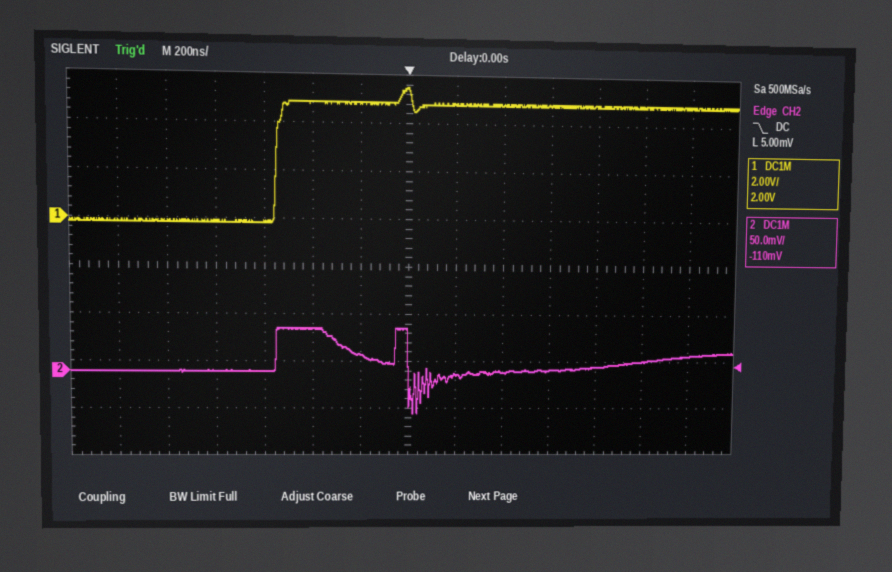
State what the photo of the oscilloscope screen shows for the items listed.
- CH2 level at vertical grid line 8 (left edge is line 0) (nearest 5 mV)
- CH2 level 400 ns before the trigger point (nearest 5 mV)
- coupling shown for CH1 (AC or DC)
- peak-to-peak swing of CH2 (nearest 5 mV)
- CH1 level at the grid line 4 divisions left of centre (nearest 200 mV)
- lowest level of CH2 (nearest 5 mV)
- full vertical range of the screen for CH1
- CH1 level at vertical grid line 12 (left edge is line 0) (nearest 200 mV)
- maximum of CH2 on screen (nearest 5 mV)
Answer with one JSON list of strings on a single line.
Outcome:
["-5 mV", "45 mV", "DC", "90 mV", "-200 mV", "-45 mV", "16 V", "4.8 V", "45 mV"]
